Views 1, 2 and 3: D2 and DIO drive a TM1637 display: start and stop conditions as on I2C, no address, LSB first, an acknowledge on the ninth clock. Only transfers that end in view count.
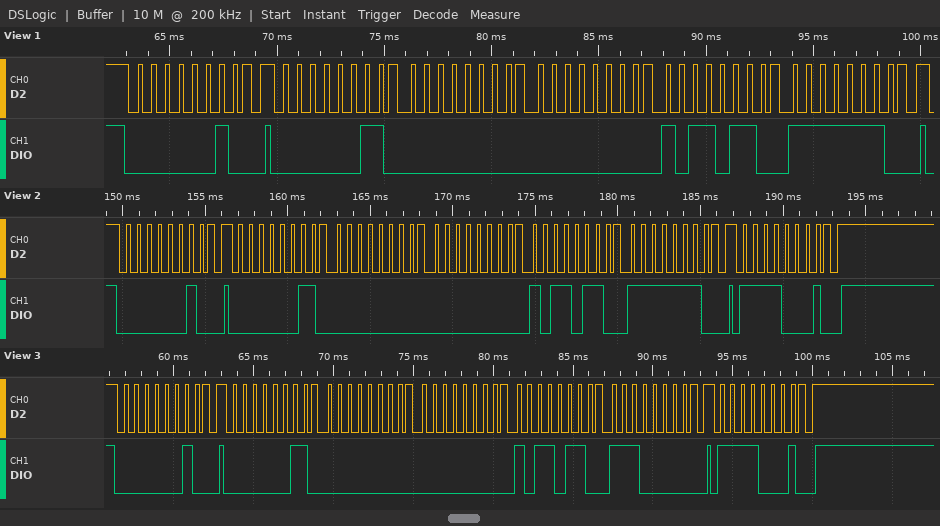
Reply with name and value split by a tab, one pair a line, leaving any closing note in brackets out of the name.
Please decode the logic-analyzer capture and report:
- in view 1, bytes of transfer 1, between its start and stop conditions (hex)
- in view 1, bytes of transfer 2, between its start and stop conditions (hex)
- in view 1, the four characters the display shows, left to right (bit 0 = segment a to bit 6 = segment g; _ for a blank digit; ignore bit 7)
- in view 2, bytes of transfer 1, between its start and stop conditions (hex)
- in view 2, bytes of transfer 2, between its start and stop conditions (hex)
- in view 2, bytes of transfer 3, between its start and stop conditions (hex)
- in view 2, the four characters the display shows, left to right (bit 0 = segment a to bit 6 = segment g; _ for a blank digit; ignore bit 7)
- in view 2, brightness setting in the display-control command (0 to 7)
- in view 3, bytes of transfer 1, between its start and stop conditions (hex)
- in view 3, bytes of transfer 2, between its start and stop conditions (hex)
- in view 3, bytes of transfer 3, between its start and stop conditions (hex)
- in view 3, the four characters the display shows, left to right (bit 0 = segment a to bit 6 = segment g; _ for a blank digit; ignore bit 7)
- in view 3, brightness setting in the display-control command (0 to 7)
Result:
in view 1, bytes of transfer 1, between its start and stop conditions	40
in view 1, bytes of transfer 2, between its start and stop conditions	C0 00 00 6D 7F
in view 1, the four characters the display shows, left to right	__58
in view 2, bytes of transfer 1, between its start and stop conditions	40
in view 2, bytes of transfer 2, between its start and stop conditions	C0 00 00 6D 7F
in view 2, bytes of transfer 3, between its start and stop conditions	8F
in view 2, the four characters the display shows, left to right	__58
in view 2, brightness setting in the display-control command	7
in view 3, bytes of transfer 1, between its start and stop conditions	40
in view 3, bytes of transfer 2, between its start and stop conditions	C0 00 00 6D 07
in view 3, bytes of transfer 3, between its start and stop conditions	8F
in view 3, the four characters the display shows, left to right	__57
in view 3, brightness setting in the display-control command	7
